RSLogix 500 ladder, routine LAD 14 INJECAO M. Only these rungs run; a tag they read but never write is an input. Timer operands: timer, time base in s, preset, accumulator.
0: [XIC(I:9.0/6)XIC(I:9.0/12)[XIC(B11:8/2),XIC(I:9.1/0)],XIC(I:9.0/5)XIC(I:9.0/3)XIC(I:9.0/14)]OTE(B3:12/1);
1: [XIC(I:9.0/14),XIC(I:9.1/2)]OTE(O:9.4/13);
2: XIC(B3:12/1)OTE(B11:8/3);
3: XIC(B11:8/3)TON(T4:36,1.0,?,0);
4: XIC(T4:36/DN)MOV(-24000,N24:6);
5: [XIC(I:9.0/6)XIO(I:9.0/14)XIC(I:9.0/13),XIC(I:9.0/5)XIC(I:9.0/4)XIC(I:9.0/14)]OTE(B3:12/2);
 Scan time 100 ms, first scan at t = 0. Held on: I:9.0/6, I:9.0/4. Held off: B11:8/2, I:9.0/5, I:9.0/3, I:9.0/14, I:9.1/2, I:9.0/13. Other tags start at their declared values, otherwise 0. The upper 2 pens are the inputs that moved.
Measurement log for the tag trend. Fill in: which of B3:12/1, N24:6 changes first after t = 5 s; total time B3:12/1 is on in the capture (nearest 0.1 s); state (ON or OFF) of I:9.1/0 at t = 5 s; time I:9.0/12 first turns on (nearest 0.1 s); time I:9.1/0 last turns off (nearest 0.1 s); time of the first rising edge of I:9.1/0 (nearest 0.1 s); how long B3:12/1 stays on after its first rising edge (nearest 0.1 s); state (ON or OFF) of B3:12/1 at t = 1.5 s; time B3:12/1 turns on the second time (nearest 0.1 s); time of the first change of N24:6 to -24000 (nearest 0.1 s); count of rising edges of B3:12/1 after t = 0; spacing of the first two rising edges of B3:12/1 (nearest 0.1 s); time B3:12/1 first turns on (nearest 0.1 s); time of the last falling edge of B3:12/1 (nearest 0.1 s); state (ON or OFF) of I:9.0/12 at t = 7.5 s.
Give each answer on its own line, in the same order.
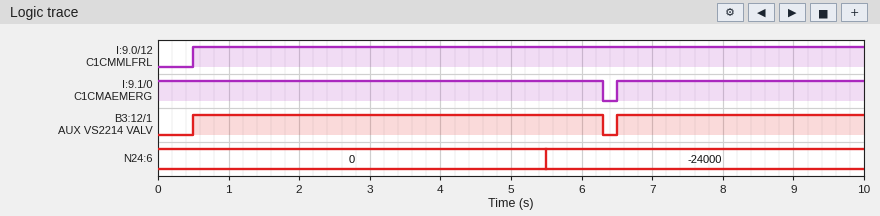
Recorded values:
N24:6
9.3 s
ON
0.5 s
6.3 s
6.5 s
5.8 s
ON
6.5 s
5.5 s
2
6.0 s
0.5 s
6.3 s
ON
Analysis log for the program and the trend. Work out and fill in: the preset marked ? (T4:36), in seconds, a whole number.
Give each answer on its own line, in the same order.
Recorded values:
5 s
